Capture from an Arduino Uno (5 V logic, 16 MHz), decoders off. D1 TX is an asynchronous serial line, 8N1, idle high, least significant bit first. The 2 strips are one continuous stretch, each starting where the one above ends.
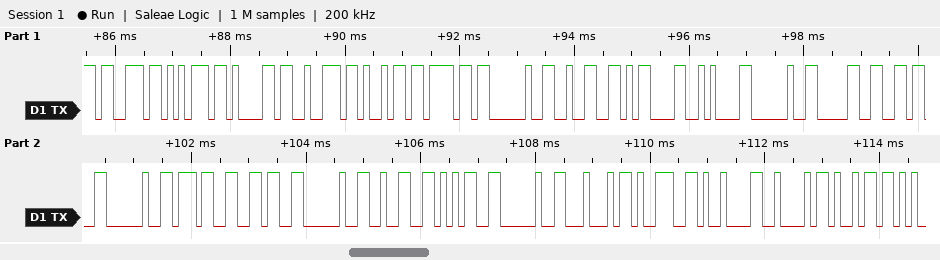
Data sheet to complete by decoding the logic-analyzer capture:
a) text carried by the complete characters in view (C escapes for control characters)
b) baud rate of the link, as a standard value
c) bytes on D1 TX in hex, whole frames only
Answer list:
"suario 2\r\n 06 76 25 D9\tBi"
9600 baud
73 75 61 72 69 6F 20 32 0D 0A 20 30 36 20 37 36 20 32 35 20 44 39 09 42 69
